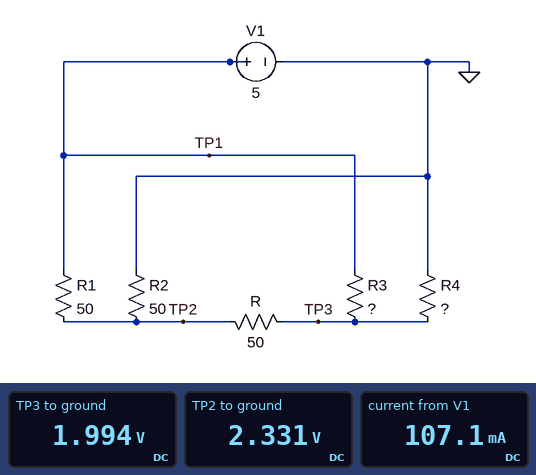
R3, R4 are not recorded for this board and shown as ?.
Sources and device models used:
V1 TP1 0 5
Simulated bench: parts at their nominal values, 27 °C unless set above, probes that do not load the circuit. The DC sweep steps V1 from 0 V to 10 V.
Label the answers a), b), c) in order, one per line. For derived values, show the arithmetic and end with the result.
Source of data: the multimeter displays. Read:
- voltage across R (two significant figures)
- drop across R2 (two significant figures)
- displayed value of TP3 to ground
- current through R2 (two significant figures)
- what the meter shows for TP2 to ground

a) 2.331 V - 1.994 V = 340 mV
b) 2.331 V = 2.3 V
c) 1.994 V
d) (2.331 V) / 50 Ω = 47 mA
e) 2.331 V
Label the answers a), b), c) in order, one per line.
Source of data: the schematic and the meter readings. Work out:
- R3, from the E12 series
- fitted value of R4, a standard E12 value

a) 56 Ω
b) 33 Ω
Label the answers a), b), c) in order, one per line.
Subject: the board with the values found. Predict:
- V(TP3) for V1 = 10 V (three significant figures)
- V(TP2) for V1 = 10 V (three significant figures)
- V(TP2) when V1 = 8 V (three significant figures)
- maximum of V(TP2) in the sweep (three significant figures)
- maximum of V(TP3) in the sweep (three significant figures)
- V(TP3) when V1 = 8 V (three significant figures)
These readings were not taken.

a) 3.99 V
b) 4.66 V
c) 3.73 V
d) 4.66 V
e) 3.99 V
f) 3.19 V
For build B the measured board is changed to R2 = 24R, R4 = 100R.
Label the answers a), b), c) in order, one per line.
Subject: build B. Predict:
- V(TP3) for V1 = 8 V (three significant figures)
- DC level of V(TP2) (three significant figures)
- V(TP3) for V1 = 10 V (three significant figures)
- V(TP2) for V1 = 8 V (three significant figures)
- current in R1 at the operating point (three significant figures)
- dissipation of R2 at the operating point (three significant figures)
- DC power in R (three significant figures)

a) 4.24 V
b) 1.87 V
c) 5.30 V
d) 3.00 V
e) 62.5 mA
f) 146 mW
g) 12.0 mW
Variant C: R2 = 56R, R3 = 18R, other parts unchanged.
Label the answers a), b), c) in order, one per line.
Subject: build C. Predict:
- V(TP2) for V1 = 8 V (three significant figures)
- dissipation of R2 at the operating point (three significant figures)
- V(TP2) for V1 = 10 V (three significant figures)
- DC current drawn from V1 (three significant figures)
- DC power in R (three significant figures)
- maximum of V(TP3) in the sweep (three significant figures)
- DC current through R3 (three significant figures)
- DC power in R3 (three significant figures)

a) 4.51 V
b) 142 mW
c) 5.64 V
d) 146 mA
e) 2.27 mW
f) 6.31 V
g) 102 mA
h) 189 mW
